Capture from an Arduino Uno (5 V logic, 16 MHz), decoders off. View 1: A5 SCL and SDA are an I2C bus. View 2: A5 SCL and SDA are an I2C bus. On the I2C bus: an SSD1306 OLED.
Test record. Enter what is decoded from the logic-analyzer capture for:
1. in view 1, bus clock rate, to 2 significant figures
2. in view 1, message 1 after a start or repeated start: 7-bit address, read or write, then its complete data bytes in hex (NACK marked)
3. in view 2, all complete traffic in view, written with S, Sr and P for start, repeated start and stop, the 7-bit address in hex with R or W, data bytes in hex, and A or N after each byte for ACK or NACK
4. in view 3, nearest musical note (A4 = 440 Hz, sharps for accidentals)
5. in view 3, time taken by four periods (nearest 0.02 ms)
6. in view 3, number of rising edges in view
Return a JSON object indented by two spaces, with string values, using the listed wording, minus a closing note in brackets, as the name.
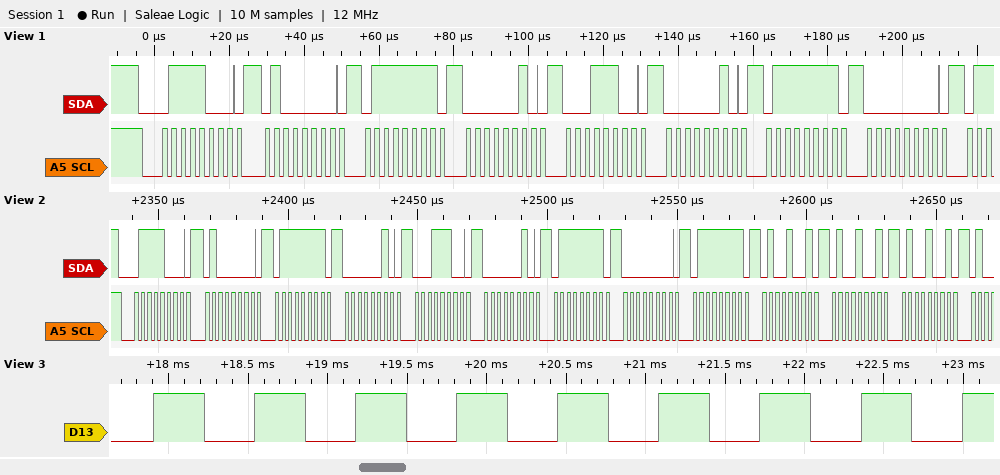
{
  "in view 1, bus clock rate, to 2 significant figures": "400 kHz",
  "in view 1, message 1 after a start or repeated start: 7-bit address, read or write, then its complete data bytes in hex": "0x3C write: 40 7F 02 1C 02 7F 00",
  "in view 2, all complete traffic in view, written with S, Sr and P for start, repeated start and stop, the 7-bit address in hex with R or W, data bytes in hex, and A or N after each byte for ACK or NACK": "S 3CW A 40 A 7F A 02 A 1C A 02 A 7F A 00 A 7F A 49 A 49 A 49 A",
  "in view 3, nearest musical note": "G6",
  "in view 3, time taken by four periods": "2.54 ms",
  "in view 3, number of rising edges in view": "9"
}
